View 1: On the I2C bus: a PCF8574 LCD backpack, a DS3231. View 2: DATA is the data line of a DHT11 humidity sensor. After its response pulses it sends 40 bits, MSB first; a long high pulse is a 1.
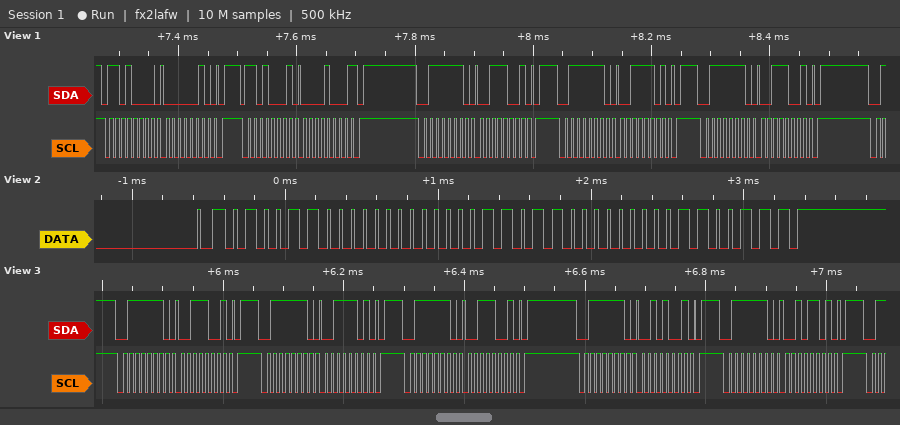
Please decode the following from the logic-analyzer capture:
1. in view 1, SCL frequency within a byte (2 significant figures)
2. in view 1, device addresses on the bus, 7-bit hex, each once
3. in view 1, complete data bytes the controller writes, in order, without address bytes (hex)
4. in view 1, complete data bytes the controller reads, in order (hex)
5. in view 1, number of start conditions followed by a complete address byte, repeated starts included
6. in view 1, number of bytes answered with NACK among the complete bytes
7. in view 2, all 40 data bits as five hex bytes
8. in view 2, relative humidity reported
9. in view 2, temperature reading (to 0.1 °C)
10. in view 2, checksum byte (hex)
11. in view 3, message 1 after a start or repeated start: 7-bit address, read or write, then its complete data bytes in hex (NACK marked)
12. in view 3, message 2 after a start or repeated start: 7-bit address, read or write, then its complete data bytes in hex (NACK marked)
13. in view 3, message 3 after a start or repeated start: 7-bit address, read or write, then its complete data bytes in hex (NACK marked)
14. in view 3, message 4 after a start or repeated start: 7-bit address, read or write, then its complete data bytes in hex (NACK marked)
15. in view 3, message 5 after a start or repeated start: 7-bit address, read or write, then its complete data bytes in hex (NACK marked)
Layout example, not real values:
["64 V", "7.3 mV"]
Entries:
["100 kHz", "0x68 0x3F", "02 39 3D 39", "08", "5", "1", "4C 00 1B 00 67", "76 %", "27.0 °C", "0x67", "0x3F write: 39", "0x3F write: 3D", "0x3F write: 39", "0x3F write: 29", "0x3F write: 2D"]
